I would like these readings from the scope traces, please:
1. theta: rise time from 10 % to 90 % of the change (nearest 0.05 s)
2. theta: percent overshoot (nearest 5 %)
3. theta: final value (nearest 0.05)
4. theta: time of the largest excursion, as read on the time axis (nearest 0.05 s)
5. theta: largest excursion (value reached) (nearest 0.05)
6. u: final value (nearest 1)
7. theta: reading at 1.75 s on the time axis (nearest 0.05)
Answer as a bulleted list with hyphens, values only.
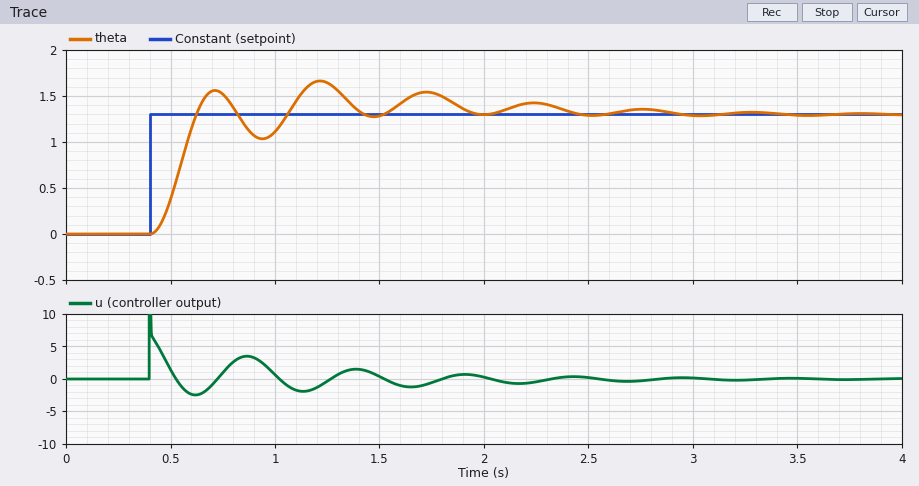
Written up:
- 0.15 s
- 30 %
- 1.30
- 1.20 s
- 1.65
- 0
- 1.55
